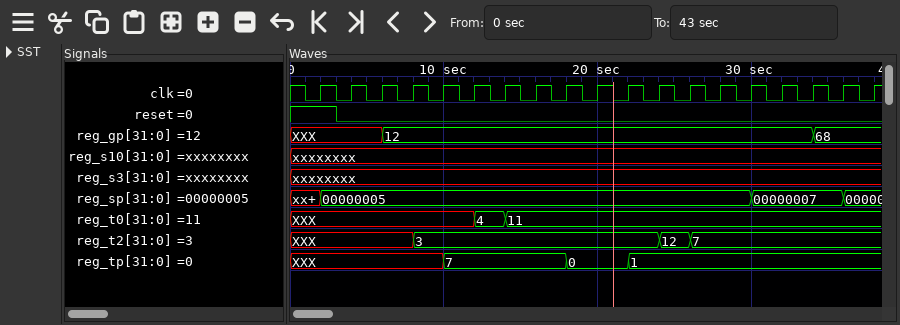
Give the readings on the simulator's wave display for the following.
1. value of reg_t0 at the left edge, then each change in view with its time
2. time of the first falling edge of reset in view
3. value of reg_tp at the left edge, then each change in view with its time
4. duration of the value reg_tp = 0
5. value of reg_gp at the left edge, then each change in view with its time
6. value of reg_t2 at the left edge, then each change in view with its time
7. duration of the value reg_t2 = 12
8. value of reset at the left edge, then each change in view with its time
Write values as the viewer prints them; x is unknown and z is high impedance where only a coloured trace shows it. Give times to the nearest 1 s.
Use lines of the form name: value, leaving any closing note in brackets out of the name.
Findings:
value of reg_t0 at the left edge, then each change in view with its time: XXX, 4 at 12 s, 11 at 14 s
time of the first falling edge of reset in view: 3 s
value of reg_tp at the left edge, then each change in view with its time: XXX, 7 at 10 s, 0 at 18 s, 1 at 22 s
duration of the value reg_tp = 0: 4 s
value of reg_gp at the left edge, then each change in view with its time: XXX, 12 at 6 s, 68 at 34 s
value of reg_t2 at the left edge, then each change in view with its time: XXX, 3 at 8 s, 12 at 24 s, 7 at 26 s
duration of the value reg_t2 = 12: 2 s
value of reset at the left edge, then each change in view with its time: 1, 0 at 3 s
